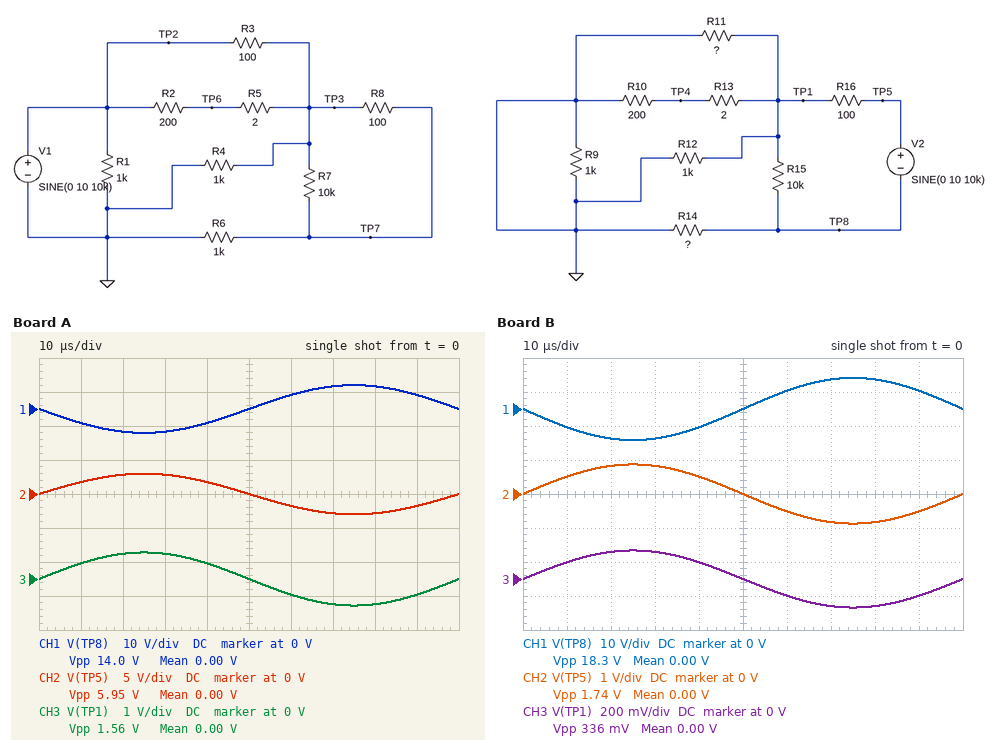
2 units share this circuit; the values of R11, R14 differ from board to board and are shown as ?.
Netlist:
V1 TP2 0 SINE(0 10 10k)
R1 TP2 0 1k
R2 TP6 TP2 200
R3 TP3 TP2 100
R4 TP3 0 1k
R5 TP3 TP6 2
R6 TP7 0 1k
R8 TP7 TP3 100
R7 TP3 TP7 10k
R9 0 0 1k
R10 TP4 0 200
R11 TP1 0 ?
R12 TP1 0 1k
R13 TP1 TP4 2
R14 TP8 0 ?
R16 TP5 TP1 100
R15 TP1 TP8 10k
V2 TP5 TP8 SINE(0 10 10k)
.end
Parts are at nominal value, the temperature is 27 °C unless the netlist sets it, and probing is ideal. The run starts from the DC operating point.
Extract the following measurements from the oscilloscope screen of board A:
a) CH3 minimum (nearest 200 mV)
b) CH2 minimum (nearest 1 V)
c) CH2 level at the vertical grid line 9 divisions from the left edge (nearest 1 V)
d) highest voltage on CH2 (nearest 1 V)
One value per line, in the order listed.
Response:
-800 mV
-3 V
-2 V
3 V
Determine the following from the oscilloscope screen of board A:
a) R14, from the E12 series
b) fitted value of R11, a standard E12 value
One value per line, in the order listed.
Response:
330 Ω
47 Ω
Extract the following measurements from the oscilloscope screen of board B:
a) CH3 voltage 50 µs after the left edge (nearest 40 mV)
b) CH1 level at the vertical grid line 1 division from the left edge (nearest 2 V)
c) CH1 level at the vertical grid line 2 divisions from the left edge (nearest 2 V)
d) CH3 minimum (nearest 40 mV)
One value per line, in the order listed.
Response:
0 V
-6 V
-8 V
-160 mV
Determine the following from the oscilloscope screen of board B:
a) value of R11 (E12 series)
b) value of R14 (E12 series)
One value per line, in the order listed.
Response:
33 Ω
1.5 kΩ
